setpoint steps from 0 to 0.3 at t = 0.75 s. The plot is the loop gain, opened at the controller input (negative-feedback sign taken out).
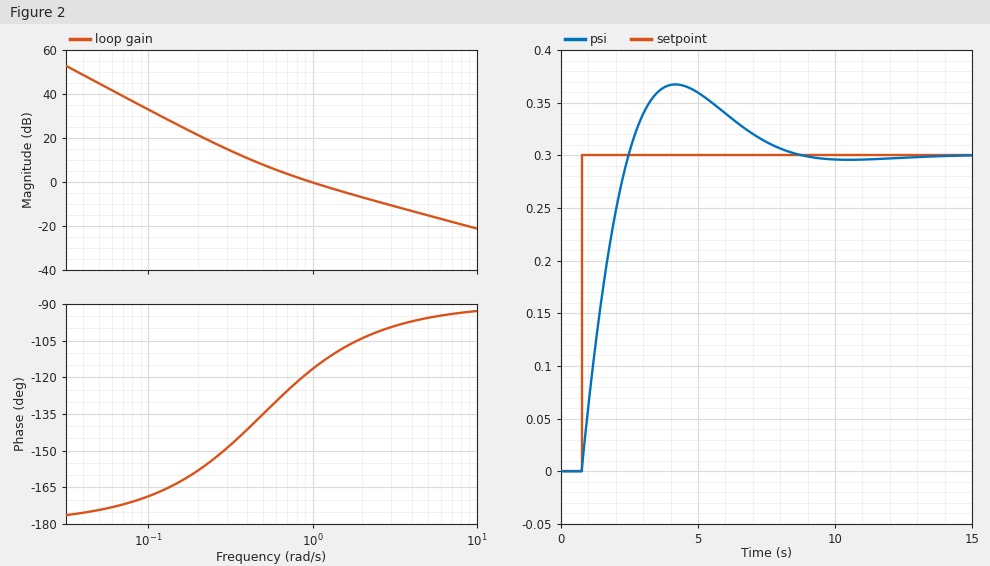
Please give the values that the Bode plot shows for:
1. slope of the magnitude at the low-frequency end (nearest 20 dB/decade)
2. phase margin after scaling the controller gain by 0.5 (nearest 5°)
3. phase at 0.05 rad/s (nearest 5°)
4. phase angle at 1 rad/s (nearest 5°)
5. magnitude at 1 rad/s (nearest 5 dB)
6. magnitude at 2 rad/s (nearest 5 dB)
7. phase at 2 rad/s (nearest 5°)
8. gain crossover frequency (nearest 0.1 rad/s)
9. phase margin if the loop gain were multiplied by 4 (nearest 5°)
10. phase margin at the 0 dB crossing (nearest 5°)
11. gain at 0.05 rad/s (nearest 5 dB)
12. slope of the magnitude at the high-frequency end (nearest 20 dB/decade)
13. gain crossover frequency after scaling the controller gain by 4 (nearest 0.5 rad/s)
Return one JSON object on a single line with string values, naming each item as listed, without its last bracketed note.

{"slope of the magnitude at the low-frequency end": "-40 dB/decade", "phase margin after scaling the controller gain by 0.5": "50°", "phase at 0.05 rad/s": "-175°", "phase angle at 1 rad/s": "-115°", "magnitude at 1 rad/s": "0 dB", "magnitude at 2 rad/s": "-5 dB", "phase at 2 rad/s": "-105°", "gain crossover frequency": "1.0 rad/s", "phase margin if the loop gain were multiplied by 4": "80°", "phase margin at the 0 dB crossing": "65°", "gain at 0.05 rad/s": "45 dB", "slope of the magnitude at the high-frequency end": "-20 dB/decade", "gain crossover frequency after scaling the controller gain by 4": "3.5 rad/s"}
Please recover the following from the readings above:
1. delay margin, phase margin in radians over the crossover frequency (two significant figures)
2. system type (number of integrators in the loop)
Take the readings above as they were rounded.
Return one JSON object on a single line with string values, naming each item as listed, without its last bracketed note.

{"delay margin, phase margin in radians over the crossover frequency": "1.1 s", "system type": "2"}
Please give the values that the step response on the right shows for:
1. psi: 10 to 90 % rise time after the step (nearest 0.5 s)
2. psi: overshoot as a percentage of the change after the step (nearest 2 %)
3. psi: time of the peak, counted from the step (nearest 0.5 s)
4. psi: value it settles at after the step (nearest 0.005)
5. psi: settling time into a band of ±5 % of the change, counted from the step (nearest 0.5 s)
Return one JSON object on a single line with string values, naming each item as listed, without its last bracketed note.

{"psi: 10 to 90 % rise time after the step": "1.5 s", "psi: overshoot as a percentage of the change after the step": "22 %", "psi: time of the peak, counted from the step": "3.5 s", "psi: value it settles at after the step": "0.300", "psi: settling time into a band of ±5 % of the change, counted from the step": "6.5 s"}
